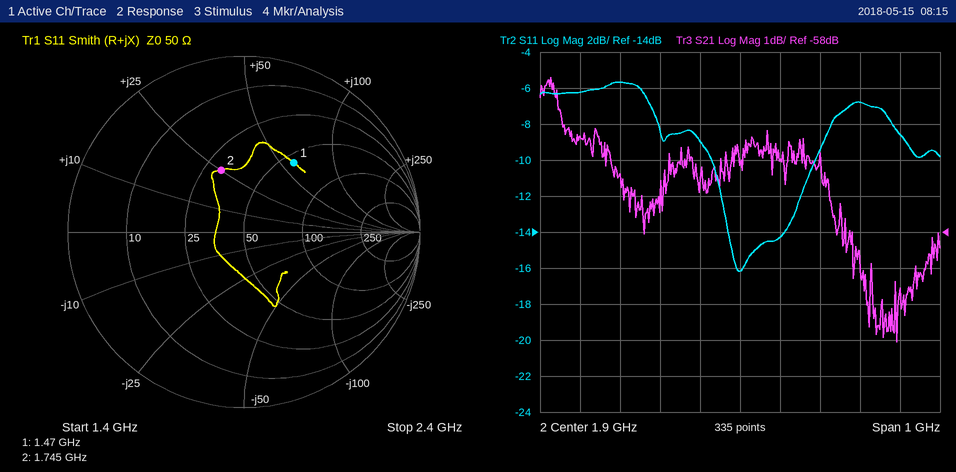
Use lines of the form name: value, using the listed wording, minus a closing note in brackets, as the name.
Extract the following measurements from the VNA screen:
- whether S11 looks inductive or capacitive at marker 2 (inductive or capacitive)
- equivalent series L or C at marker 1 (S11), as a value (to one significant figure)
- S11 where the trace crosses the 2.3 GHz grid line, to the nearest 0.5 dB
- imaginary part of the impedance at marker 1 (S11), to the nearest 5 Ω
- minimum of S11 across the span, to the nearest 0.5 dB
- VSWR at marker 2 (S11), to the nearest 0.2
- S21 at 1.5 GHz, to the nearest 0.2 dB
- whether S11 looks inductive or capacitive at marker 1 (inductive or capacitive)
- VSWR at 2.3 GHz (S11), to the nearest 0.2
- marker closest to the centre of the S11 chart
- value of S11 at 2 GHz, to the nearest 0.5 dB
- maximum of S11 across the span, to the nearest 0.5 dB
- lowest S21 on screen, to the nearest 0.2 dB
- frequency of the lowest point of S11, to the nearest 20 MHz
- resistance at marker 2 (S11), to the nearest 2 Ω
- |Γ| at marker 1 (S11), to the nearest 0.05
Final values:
whether S11 looks inductive or capacitive at marker 2: inductive
equivalent series L or C at marker 1 (S11), as a value: 6 nH
S11 where the trace crosses the 2.3 GHz grid line, to the nearest 0.5 dB: -8.5 dB
imaginary part of the impedance at marker 1 (S11), to the nearest 5 Ω: +60 Ω
minimum of S11 across the span, to the nearest 0.5 dB: -16.0 dB
VSWR at marker 2 (S11), to the nearest 0.2: 2.2
S21 at 1.5 GHz, to the nearest 0.2 dB: -55.4 dB
whether S11 looks inductive or capacitive at marker 1: inductive
VSWR at 2.3 GHz (S11), to the nearest 0.2: 2.2
marker closest to the centre of the S11 chart: marker 2
value of S11 at 2 GHz, to the nearest 0.5 dB: -14.5 dB
maximum of S11 across the span, to the nearest 0.5 dB: -5.5 dB
lowest S21 on screen, to the nearest 0.2 dB: -61.0 dB
frequency of the lowest point of S11, to the nearest 20 MHz: 1.90 GHz
resistance at marker 2 (S11), to the nearest 2 Ω: 30 Ω
|Γ| at marker 1 (S11), to the nearest 0.05: 0.50
